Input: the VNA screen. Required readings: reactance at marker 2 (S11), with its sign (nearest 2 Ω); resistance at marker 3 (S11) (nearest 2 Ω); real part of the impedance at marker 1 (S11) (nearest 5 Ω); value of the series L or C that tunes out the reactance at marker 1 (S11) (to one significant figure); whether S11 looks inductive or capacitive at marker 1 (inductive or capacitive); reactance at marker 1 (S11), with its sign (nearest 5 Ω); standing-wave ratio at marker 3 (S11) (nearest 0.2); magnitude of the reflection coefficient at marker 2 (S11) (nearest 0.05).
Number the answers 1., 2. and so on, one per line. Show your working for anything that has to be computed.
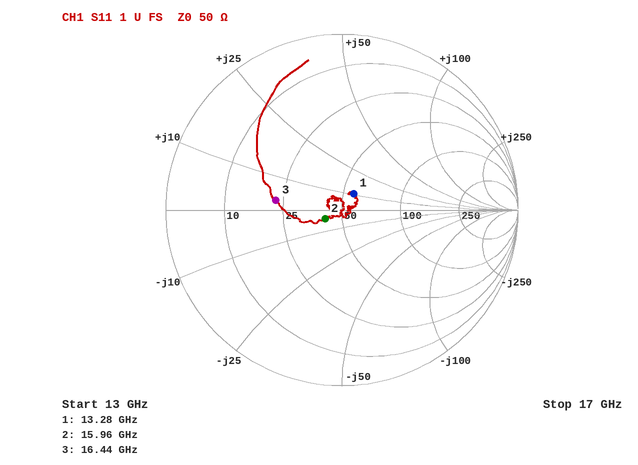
1. -4 Ω
2. 22 Ω
3. 55 Ω
4. C = 1/(2π × 13.28 GHz × 10 Ω) ≈ 1 pF
5. inductive
6. +10 Ω
7. 2.2
8. 0.10
